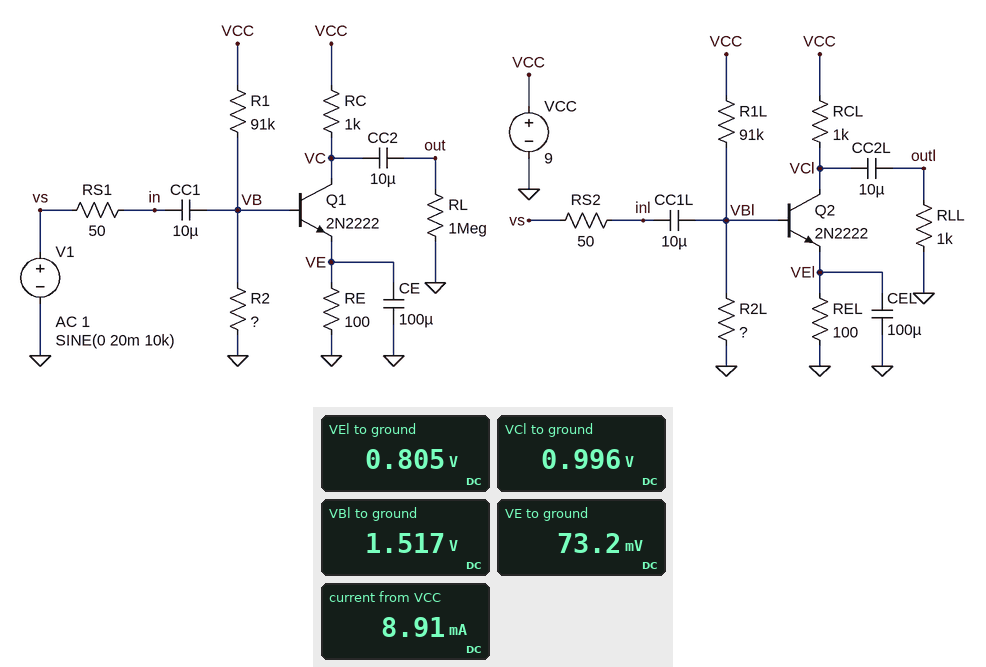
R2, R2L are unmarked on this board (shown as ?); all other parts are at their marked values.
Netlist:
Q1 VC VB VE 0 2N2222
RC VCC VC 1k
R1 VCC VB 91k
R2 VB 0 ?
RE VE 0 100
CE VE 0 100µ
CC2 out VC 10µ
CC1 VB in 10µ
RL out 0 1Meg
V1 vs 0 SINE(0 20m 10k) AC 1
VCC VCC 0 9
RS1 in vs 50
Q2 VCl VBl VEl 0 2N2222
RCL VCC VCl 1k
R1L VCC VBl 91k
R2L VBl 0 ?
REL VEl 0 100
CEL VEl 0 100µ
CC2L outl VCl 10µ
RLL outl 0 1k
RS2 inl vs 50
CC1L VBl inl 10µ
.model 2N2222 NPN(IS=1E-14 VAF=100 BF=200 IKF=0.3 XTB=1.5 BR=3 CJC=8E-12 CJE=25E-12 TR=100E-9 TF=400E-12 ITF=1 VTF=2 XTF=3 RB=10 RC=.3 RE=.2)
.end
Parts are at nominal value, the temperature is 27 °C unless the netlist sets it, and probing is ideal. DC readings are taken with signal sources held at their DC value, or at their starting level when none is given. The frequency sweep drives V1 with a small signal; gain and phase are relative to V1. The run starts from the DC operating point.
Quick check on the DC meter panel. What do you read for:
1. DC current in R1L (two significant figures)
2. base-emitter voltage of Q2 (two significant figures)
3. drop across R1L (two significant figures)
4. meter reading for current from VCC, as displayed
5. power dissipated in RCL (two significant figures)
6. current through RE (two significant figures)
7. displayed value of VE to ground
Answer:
82 µA
710 mV
7.5 V
8.91 mA
64 mW
730 µA
73.2 mV
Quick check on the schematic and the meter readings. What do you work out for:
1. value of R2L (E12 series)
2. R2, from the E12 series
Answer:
39 kΩ
8.2 kΩ
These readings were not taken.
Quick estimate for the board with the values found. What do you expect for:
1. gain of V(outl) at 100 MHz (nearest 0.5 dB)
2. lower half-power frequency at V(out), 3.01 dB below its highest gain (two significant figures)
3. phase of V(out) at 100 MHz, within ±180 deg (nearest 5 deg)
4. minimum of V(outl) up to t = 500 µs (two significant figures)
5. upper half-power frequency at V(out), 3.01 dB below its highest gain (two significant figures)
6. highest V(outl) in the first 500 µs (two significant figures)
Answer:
-3.5 dB
57 Hz
65 deg
-150 mV
13 MHz
1.9 V
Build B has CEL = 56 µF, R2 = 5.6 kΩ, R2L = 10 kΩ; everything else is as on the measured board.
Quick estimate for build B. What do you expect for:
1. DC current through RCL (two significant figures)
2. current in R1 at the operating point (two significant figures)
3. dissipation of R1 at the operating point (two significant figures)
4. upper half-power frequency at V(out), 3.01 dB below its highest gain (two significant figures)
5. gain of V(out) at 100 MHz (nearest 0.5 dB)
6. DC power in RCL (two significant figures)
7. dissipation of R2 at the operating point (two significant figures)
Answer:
1.6 mA
93 µA
790 µW
150 MHz
-5.5 dB
2.5 mW
49 µW
